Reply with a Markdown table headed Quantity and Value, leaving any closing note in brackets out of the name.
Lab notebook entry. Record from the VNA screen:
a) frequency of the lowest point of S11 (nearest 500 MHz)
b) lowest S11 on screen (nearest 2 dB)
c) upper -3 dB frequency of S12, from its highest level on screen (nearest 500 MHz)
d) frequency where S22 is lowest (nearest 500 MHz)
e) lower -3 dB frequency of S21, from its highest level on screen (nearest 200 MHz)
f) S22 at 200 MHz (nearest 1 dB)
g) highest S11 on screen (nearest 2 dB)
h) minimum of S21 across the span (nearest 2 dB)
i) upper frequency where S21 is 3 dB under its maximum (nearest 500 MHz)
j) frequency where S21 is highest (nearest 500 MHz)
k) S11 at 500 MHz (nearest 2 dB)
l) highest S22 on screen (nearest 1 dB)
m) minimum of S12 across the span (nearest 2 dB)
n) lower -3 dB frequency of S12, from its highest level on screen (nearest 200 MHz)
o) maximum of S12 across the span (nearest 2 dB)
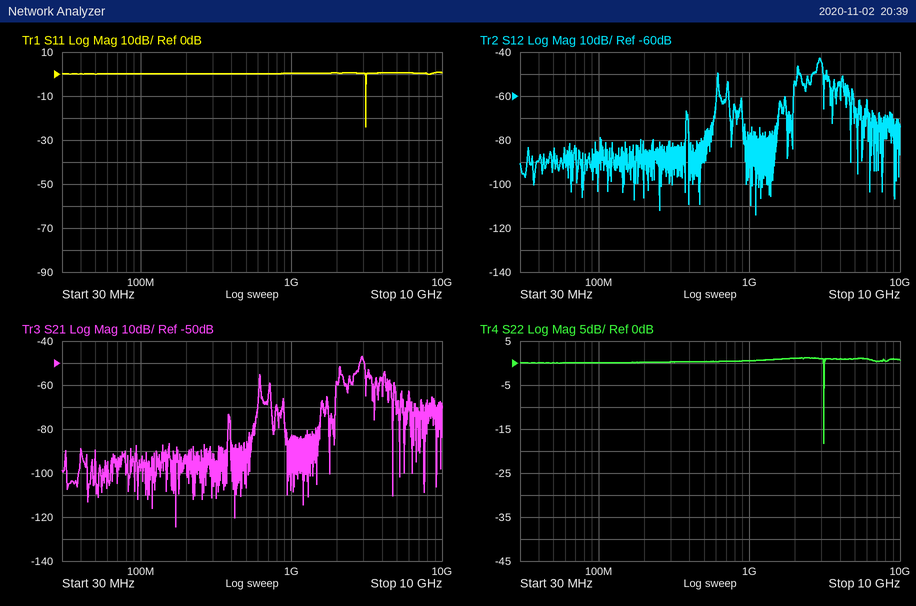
| Quantity | Value |
|---|---|
| frequency of the lowest point of S11 | 3.0 GHz |
| lowest S11 on screen | -24 dB |
| upper -3 dB frequency of S12, from its highest level on screen | 3.0 GHz |
| frequency where S22 is lowest | 3.0 GHz |
| lower -3 dB frequency of S21, from its highest level on screen | 2.8 GHz |
| S22 at 200 MHz | 0 dB |
| highest S11 on screen | 0 dB |
| minimum of S21 across the span | -124 dB |
| upper frequency where S21 is 3 dB under its maximum | 3.0 GHz |
| frequency where S21 is highest | 3.0 GHz |
| S11 at 500 MHz | 0 dB |
| highest S22 on screen | 1 dB |
| minimum of S12 across the span | -114 dB |
| lower -3 dB frequency of S12, from its highest level on screen | 2.8 GHz |
| maximum of S12 across the span | -42 dB |
